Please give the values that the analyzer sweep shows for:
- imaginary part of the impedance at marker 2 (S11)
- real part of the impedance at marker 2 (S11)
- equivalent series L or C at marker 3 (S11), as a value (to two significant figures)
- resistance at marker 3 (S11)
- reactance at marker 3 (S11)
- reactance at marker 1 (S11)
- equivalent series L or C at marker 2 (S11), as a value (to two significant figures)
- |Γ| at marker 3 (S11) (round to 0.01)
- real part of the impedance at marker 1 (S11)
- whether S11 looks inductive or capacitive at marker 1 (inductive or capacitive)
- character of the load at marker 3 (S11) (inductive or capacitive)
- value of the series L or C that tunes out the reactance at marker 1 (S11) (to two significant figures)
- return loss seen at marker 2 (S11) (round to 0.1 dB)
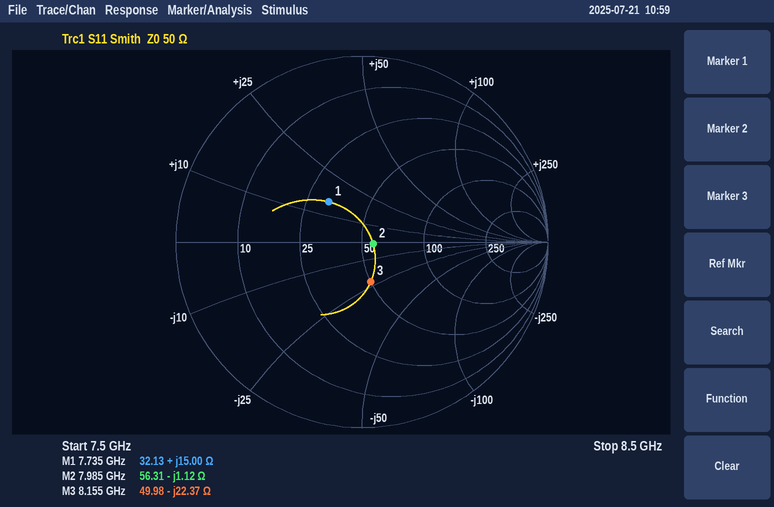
-1.12 Ω
56.31 Ω
870 fF
49.98 Ω
-22.37 Ω
+15.00 Ω
18 pF
0.22
32.13 Ω
inductive
capacitive
1.4 pF
24.4 dB
